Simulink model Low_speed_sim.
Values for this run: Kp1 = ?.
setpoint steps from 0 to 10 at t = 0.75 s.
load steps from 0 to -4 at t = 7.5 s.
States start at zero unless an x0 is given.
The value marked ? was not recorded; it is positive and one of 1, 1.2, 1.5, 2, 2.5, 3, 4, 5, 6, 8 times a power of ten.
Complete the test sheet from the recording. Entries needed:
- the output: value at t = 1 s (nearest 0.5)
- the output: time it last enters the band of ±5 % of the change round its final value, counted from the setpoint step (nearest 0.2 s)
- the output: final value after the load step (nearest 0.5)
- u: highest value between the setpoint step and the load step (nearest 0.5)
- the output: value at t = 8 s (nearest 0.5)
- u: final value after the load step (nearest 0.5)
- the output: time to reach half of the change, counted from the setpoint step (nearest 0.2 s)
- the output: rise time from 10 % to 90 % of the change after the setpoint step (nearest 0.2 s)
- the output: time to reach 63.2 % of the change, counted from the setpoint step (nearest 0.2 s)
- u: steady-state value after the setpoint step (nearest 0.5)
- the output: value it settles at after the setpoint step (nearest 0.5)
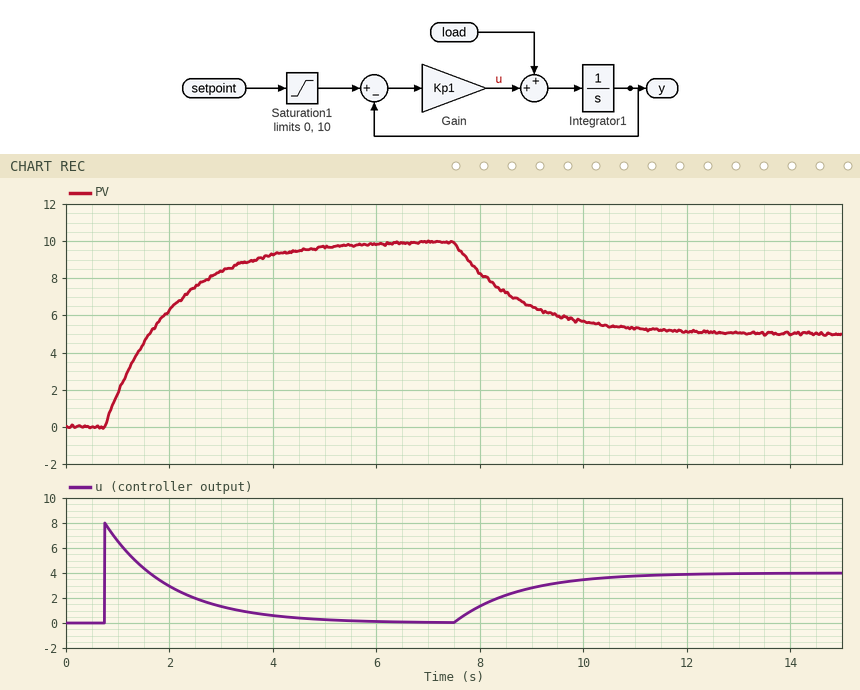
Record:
2.0
3.8 s
5.0
8.0
8.5
4.0
0.8 s
2.8 s
1.2 s
0.0
10.0
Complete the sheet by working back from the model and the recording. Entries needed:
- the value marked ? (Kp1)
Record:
0.8
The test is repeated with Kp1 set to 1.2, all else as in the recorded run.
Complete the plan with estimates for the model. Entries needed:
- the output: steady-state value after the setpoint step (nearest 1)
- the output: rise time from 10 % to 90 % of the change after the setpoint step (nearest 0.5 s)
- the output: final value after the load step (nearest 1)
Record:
10
2.0 s
7
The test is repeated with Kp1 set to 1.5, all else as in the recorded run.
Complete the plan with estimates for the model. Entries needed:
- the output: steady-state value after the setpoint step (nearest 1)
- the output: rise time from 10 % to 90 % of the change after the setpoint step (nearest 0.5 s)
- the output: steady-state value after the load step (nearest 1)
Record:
10
1.5 s
7
